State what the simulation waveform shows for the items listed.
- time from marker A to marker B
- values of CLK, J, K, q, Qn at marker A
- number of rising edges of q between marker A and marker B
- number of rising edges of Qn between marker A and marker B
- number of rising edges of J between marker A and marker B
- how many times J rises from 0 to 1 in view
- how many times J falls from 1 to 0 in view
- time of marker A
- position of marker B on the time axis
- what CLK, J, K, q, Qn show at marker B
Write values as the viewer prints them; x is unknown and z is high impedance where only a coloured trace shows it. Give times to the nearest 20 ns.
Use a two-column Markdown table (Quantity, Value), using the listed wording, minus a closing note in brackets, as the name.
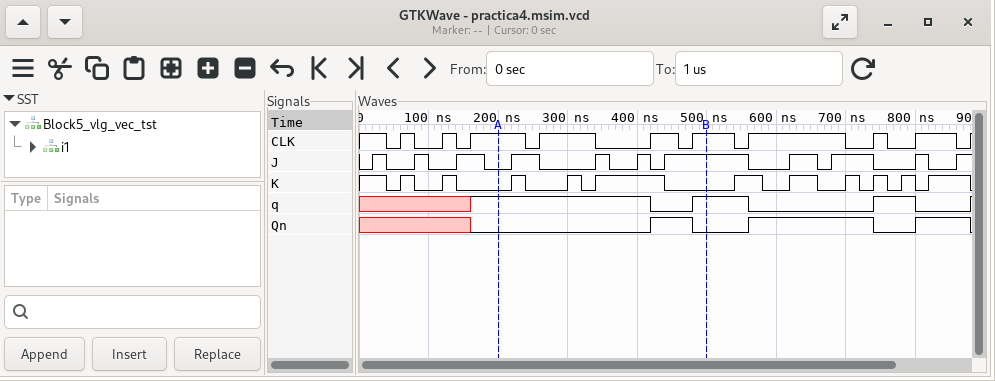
| Quantity | Value |
|---|---|
| time from marker A to marker B | 300 ns |
| values of CLK, J, K, q, Qn at marker A | CLK=1, J=0, K=0, q=1, Qn=0 |
| number of rising edges of q between marker A and marker B | 1 |
| number of rising edges of Qn between marker A and marker B | 1 |
| number of rising edges of J between marker A and marker B | 4 |
| how many times J rises from 0 to 1 in view | 11 |
| how many times J falls from 1 to 0 in view | 10 |
| time of marker A | 200 ns |
| position of marker B on the time axis | 500 ns |
| what CLK, J, K, q, Qn show at marker B | CLK=1, J=1, K=0, q=1, Qn=0 |
